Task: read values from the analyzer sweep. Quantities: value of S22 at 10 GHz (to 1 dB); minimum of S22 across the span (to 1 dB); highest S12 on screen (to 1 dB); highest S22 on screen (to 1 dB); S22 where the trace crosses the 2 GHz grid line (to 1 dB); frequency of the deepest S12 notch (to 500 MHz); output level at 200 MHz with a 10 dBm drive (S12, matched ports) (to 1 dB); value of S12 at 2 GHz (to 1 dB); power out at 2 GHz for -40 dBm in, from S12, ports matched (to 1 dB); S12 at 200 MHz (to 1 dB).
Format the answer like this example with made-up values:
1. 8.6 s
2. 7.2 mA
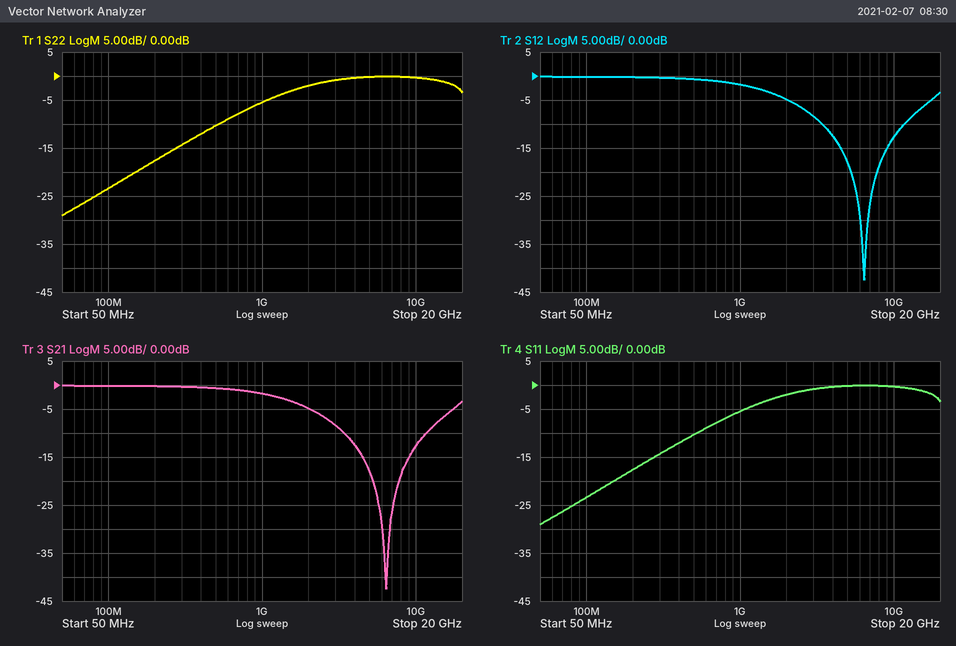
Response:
1. 0 dB
2. -29 dB
3. 0 dB
4. 0 dB
5. -2 dB
6. 6.5 GHz
7. 10 dBm
8. -5 dB
9. -45 dBm
10. 0 dB
